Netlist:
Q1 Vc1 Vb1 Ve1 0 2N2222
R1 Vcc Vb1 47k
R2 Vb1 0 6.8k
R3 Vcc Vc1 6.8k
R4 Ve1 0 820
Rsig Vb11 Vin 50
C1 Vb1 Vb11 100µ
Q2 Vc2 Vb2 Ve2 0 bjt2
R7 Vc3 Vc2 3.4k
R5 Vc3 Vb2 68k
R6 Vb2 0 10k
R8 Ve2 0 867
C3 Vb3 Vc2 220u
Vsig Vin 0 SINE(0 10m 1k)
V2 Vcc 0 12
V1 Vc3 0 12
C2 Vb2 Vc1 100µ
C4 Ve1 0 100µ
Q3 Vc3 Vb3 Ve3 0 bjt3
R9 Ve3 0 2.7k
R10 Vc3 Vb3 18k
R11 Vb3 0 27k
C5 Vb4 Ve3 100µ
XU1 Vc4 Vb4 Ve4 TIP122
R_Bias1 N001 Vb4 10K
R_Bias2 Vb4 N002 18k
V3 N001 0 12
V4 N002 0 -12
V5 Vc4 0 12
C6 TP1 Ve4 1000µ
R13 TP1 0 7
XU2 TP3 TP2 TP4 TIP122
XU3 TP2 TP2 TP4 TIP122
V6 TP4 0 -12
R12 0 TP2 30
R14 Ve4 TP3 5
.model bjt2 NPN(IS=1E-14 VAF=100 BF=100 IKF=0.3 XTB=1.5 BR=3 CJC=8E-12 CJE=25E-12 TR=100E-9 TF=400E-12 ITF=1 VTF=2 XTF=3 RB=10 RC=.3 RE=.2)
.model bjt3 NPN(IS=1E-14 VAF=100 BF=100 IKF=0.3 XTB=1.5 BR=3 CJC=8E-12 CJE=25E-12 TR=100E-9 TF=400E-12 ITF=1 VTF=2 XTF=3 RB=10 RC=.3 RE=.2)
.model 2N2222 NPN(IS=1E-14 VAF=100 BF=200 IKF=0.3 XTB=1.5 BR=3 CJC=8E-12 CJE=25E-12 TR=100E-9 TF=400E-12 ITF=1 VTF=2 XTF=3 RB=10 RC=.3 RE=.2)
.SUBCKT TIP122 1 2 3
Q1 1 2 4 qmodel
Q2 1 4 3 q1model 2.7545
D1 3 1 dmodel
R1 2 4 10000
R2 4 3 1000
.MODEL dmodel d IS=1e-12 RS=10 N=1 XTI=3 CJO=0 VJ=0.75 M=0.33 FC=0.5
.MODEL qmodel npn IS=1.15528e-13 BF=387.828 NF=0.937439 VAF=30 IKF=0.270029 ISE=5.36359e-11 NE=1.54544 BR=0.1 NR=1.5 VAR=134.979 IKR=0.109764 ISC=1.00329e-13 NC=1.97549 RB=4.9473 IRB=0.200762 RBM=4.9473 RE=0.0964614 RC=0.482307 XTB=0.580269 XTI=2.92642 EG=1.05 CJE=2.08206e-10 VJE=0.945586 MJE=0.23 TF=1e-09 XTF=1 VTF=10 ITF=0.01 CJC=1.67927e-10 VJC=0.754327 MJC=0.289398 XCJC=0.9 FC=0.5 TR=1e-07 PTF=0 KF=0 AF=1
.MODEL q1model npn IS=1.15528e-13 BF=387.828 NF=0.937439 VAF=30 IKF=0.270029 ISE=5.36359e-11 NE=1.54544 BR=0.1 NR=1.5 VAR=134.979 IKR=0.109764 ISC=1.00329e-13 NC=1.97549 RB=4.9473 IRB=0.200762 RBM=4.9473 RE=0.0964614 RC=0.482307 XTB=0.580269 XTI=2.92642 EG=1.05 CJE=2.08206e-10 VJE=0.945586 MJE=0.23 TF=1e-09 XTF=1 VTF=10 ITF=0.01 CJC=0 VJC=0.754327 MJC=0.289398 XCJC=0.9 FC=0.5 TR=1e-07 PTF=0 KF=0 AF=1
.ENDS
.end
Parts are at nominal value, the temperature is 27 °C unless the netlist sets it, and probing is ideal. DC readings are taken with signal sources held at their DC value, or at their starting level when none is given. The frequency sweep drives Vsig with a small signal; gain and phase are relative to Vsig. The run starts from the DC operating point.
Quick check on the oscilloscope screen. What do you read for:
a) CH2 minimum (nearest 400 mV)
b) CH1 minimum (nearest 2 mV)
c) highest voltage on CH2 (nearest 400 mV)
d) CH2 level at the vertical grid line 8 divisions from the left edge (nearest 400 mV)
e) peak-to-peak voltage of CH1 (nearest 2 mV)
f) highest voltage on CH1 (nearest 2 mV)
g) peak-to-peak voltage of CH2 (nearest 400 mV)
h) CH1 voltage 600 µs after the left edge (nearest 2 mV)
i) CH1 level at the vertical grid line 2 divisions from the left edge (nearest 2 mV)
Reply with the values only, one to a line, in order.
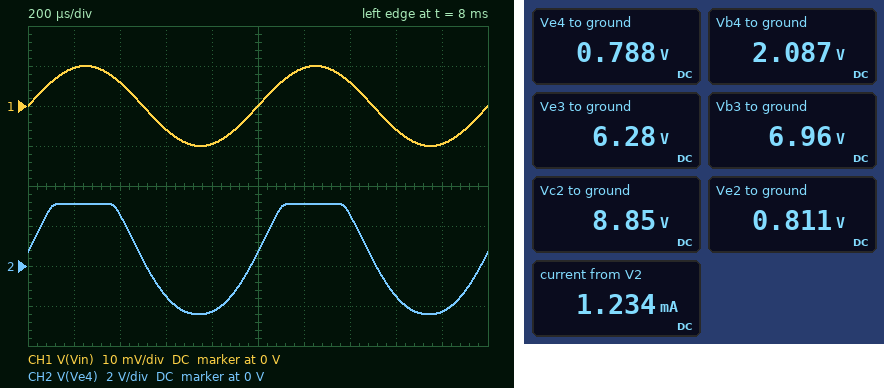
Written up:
-2.4 V
-10 mV
3.2 V
-1.6 V
20 mV
10 mV
5.6 V
-6 mV
6 mV
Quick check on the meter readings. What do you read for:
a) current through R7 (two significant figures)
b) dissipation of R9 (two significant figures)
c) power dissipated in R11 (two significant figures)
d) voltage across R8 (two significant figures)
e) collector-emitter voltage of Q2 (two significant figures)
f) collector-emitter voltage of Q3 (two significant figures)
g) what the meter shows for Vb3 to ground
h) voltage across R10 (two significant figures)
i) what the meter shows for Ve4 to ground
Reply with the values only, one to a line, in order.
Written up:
930 µA
15 mW
1.8 mW
810 mV
8.0 V
5.7 V
6.96 V
5.0 V
0.788 V
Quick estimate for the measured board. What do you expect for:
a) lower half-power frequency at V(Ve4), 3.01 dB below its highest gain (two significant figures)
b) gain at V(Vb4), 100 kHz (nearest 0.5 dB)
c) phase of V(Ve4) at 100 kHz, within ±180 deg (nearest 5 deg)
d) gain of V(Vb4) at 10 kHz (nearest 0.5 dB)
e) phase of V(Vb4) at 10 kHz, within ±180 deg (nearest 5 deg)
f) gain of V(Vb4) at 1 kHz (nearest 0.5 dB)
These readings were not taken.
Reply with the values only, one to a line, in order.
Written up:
61 Hz
51.5 dB
-5 deg
51.5 dB
0 deg
51.5 dB
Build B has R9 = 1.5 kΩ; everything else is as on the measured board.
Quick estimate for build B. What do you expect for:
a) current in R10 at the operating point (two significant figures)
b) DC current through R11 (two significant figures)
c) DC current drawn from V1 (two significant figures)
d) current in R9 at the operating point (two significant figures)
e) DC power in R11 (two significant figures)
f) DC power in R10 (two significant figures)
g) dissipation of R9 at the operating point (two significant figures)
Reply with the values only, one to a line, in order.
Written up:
290 µA
250 µA
5.4 mA
4.1 mA
1.7 mW
1.5 mW
25 mW
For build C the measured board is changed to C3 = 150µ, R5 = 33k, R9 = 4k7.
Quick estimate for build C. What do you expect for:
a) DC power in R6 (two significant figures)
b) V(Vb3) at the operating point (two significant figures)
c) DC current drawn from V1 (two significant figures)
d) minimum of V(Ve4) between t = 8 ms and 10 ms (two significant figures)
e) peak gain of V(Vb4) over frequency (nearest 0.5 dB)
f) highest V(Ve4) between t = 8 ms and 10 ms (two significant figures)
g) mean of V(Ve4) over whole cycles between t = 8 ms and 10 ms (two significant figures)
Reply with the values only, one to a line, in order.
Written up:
690 µW
7.1 V
4.1 mA
-910 mV
51.0 dB
4.6 V
1.2 V
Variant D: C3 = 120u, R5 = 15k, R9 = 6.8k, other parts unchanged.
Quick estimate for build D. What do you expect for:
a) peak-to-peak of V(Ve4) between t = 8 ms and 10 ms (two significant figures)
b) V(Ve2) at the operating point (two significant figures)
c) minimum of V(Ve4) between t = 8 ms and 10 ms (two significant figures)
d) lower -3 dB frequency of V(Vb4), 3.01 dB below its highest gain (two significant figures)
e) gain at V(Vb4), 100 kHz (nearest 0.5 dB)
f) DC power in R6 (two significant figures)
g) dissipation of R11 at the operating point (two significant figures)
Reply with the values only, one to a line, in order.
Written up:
1.1 V
2.6 V
700 mV
89 Hz
25.0 dB
1.1 mW
1.9 mW
